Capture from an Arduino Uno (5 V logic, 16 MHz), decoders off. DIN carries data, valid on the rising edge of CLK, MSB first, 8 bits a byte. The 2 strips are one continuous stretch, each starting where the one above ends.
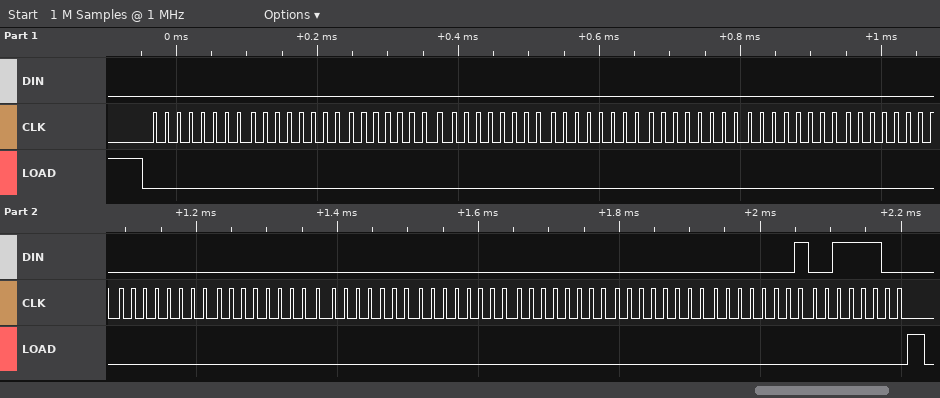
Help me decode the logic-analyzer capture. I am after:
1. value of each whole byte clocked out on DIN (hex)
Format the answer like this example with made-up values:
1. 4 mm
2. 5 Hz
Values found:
1. 00 00 00 00 00 00 00 00 00 00 00 00 00 00 01 3C
